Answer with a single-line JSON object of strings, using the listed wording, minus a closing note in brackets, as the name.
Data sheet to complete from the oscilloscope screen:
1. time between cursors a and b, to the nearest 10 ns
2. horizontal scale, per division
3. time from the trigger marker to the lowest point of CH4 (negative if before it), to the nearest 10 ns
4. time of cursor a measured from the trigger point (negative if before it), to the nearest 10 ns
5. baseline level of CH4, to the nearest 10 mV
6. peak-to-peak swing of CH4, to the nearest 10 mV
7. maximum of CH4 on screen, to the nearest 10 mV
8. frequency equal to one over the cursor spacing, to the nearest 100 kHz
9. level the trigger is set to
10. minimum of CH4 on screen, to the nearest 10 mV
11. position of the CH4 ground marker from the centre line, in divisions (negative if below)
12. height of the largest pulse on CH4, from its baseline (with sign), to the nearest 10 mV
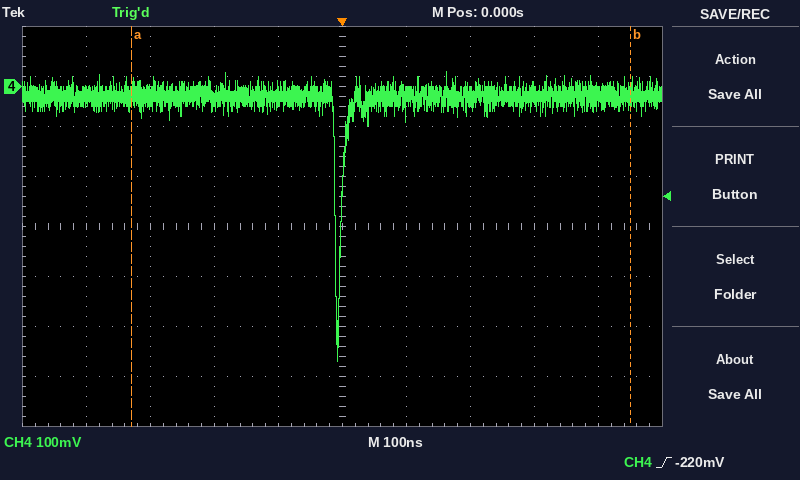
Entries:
{"time between cursors a and b, to the nearest 10 ns": "780 ns", "horizontal scale, per division": "100 ns", "time from the trigger marker to the lowest point of CH4 (negative if before it), to the nearest 10 ns": "-10 ns", "time of cursor a measured from the trigger point (negative if before it), to the nearest 10 ns": "-330 ns", "baseline level of CH4, to the nearest 10 mV": "-20 mV", "peak-to-peak swing of CH4, to the nearest 10 mV": "580 mV", "maximum of CH4 on screen, to the nearest 10 mV": "30 mV", "frequency equal to one over the cursor spacing, to the nearest 100 kHz": "1.3 MHz", "level the trigger is set to": "-220 mV", "minimum of CH4 on screen, to the nearest 10 mV": "-550 mV", "position of the CH4 ground marker from the centre line, in divisions": "+2.8 div", "height of the largest pulse on CH4, from its baseline (with sign), to the nearest 10 mV": "-530 mV"}
